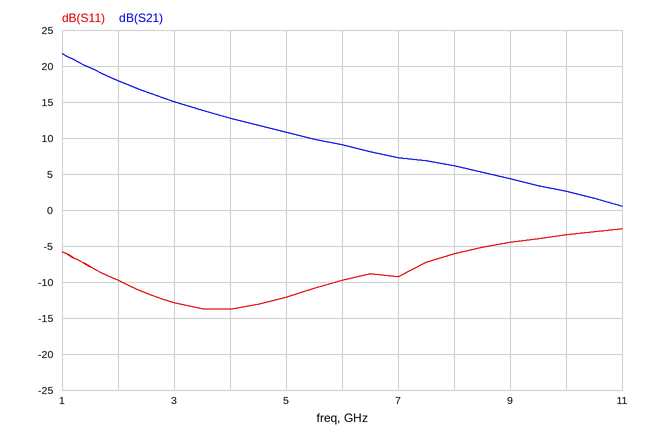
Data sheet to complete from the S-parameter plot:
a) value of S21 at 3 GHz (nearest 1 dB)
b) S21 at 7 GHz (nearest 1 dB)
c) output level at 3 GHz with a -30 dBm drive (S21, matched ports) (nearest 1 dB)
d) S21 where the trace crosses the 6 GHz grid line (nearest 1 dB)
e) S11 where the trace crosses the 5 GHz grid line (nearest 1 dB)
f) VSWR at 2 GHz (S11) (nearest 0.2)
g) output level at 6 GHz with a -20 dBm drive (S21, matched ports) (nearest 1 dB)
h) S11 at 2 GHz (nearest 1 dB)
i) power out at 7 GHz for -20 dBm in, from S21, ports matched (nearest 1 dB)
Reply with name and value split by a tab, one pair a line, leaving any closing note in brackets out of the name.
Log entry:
value of S21 at 3 GHz	15 dB
S21 at 7 GHz	7 dB
output level at 3 GHz with a -30 dBm drive (S21, matched ports)	-15 dBm
S21 where the trace crosses the 6 GHz grid line	9 dB
S11 where the trace crosses the 5 GHz grid line	-12 dB
VSWR at 2 GHz (S11)	2.0
output level at 6 GHz with a -20 dBm drive (S21, matched ports)	-11 dBm
S11 at 2 GHz	-10 dB
power out at 7 GHz for -20 dBm in, from S21, ports matched	-13 dBm
